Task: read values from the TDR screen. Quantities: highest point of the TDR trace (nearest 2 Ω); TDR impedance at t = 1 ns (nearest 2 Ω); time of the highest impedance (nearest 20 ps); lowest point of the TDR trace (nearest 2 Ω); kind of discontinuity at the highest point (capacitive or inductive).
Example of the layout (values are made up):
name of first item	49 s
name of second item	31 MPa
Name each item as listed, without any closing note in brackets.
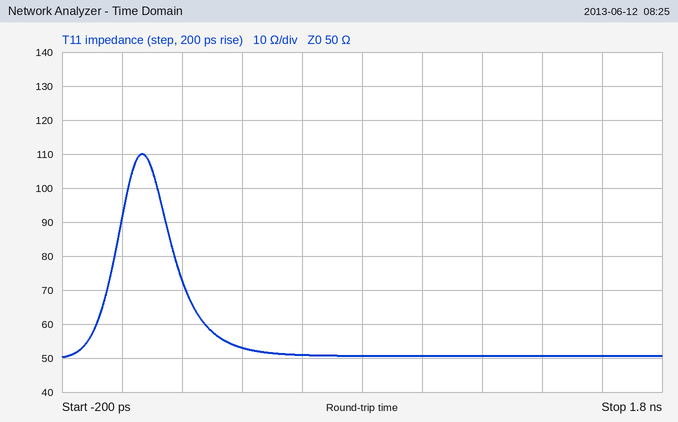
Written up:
highest point of the TDR trace	110 Ω
TDR impedance at t = 1 ns	50 Ω
time of the highest impedance	60 ps
lowest point of the TDR trace	50 Ω
kind of discontinuity at the highest point	inductive
